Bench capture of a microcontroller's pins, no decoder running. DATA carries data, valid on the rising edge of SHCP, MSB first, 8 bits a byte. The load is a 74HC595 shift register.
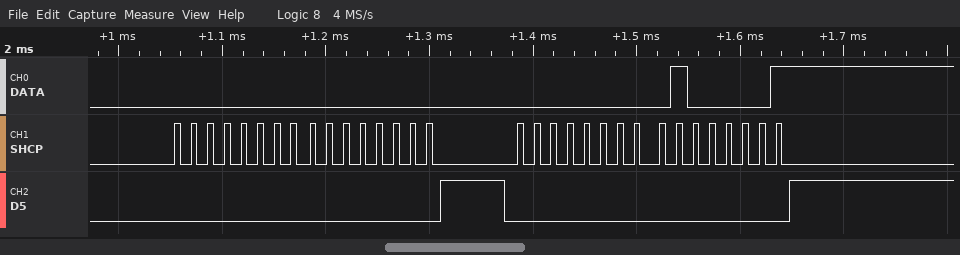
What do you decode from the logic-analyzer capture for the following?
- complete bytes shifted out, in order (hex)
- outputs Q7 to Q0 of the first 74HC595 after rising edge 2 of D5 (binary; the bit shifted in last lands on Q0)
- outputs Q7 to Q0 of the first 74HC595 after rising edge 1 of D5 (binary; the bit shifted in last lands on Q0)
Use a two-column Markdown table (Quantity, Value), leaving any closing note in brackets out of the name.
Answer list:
| Quantity | Value |
|---|---|
| complete bytes shifted out, in order | 00 00 00 41 |
| outputs Q7 to Q0 of the first 74HC595 after rising edge 2 of D5 | 01000001 |
| outputs Q7 to Q0 of the first 74HC595 after rising edge 1 of D5 | 00000000 |
